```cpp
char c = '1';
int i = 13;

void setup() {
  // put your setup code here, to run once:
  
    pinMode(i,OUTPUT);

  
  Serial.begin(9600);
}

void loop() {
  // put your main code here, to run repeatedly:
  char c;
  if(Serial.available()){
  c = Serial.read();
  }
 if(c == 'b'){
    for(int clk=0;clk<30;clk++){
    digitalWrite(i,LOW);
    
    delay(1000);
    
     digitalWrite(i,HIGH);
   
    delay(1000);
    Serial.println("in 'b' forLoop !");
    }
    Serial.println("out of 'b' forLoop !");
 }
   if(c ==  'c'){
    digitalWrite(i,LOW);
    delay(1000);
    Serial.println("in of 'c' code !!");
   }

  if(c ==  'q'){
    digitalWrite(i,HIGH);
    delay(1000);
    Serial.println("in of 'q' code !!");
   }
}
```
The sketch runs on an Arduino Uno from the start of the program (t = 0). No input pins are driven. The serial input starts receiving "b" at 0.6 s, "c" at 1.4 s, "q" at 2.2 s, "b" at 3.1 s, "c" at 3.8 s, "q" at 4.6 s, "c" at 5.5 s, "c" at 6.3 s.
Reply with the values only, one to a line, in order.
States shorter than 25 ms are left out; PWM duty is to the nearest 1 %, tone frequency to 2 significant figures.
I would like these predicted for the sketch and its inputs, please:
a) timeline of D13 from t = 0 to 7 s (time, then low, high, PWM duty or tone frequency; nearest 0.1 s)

0 s low; 1.6 s high; 2.6 s low; 3.6 s high; 4.6 s low; 5.6 s high; 6.6 s low
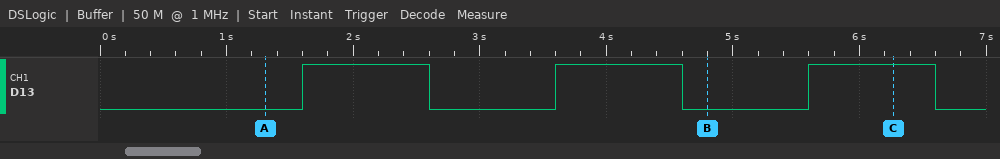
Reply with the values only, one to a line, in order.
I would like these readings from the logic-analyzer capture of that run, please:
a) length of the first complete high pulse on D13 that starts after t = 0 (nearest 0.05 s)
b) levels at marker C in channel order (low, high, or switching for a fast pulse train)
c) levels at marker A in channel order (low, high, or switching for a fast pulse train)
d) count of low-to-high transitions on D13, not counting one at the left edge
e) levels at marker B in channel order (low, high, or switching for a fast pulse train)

1.00 s
D13 high
D13 low
3
D13 low
